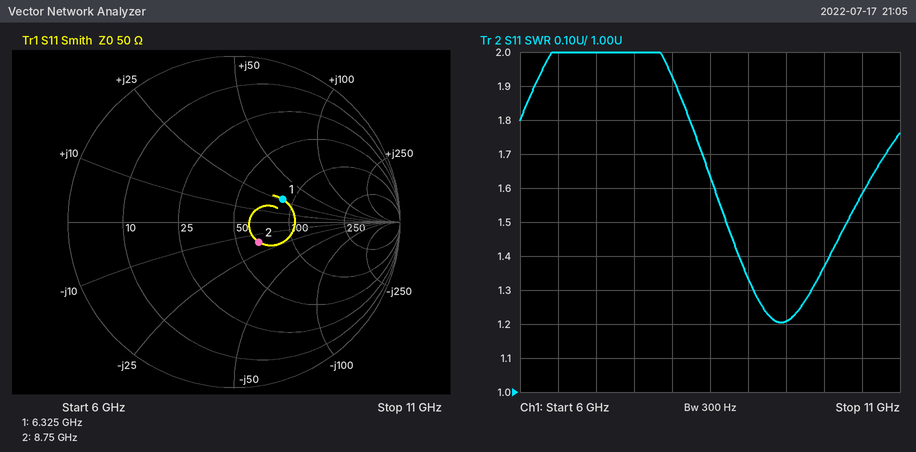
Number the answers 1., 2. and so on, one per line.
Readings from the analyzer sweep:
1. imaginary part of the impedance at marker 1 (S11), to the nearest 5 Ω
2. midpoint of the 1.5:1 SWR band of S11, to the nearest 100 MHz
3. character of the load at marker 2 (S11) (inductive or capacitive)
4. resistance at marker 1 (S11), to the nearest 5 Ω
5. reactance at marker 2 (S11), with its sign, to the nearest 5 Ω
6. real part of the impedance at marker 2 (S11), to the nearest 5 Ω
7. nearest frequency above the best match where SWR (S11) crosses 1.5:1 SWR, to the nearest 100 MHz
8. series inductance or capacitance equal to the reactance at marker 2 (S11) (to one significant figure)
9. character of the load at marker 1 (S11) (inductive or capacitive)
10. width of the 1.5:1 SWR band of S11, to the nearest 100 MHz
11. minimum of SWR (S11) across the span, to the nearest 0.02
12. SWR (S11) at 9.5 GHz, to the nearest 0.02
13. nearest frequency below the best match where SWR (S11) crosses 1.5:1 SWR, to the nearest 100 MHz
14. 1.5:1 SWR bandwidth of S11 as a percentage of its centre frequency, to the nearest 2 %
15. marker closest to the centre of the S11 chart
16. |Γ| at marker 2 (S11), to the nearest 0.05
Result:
1. +25 Ω
2. 9.5 GHz
3. capacitive
4. 85 Ω
5. -15 Ω
6. 65 Ω
7. 10.3 GHz
8. 1 pF
9. inductive
10. 1.6 GHz
11. 1.20
12. 1.20
13. 8.7 GHz
14. 16 %
15. marker 2
16. 0.20
